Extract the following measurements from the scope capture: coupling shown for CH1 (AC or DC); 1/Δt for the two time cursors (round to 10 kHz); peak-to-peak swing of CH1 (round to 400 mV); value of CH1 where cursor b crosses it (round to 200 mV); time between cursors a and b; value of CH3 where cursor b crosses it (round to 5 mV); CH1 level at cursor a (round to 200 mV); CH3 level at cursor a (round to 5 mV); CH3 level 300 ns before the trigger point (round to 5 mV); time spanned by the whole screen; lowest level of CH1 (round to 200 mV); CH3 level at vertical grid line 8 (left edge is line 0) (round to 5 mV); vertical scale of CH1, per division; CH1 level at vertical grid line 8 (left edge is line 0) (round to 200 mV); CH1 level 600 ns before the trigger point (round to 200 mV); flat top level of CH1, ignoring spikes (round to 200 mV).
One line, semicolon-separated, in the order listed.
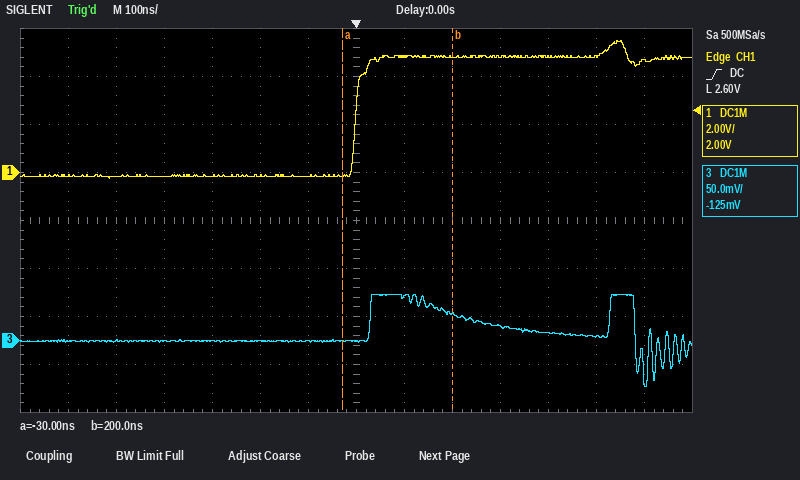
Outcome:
DC; 4.35 MHz; 5.6 V; 4.8 V; 230 ns; 30 mV; -200 mV; 0 mV; 0 mV; 1.4 µs; -200 mV; 45 mV; 2 V; 4.8 V; -200 mV; 4.8 V
